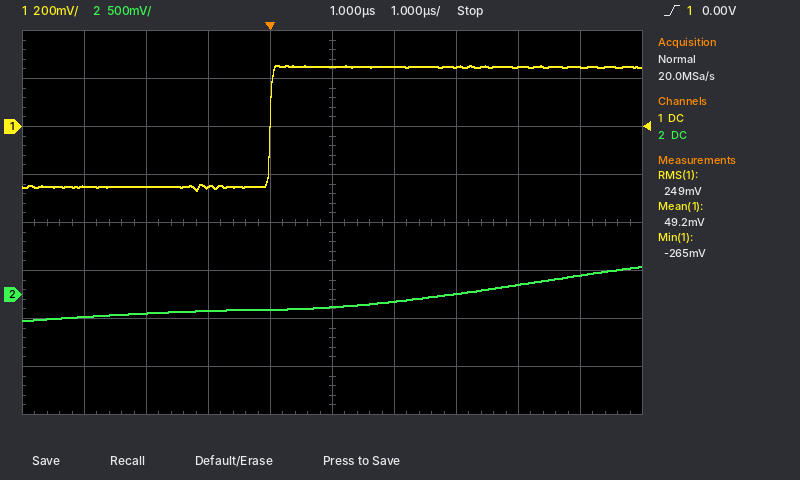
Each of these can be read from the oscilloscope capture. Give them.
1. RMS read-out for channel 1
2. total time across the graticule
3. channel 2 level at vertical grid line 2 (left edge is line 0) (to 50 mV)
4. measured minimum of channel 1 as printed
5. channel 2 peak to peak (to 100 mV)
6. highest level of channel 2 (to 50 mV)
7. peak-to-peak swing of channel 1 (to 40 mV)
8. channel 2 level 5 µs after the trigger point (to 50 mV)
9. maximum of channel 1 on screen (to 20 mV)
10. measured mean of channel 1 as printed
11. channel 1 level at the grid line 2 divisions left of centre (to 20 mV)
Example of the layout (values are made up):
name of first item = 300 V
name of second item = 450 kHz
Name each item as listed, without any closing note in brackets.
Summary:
RMS read-out for channel 1 = 249 mV
total time across the graticule = 10 µs
channel 2 level at vertical grid line 2 (left edge is line 0) = -200 mV
measured minimum of channel 1 as printed = -265 mV
channel 2 peak to peak = 600 mV
highest level of channel 2 = 300 mV
peak-to-peak swing of channel 1 = 520 mV
channel 2 level 5 µs after the trigger point = 200 mV
maximum of channel 1 on screen = 260 mV
measured mean of channel 1 as printed = 49.2 mV
channel 1 level at the grid line 2 divisions left of centre = -260 mV
